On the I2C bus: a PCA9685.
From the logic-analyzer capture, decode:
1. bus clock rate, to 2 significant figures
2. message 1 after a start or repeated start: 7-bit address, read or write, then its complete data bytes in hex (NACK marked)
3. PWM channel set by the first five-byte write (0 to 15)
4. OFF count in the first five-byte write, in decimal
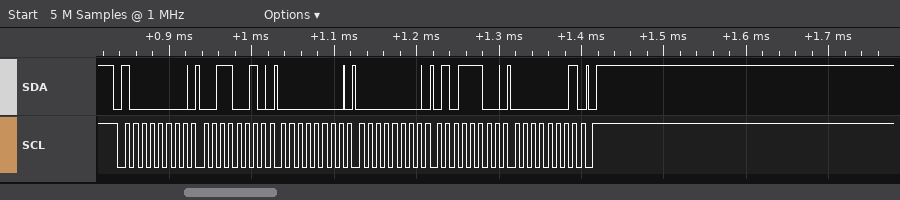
100 kHz
0x40 write: 32 00 00 5C 01
11
348
